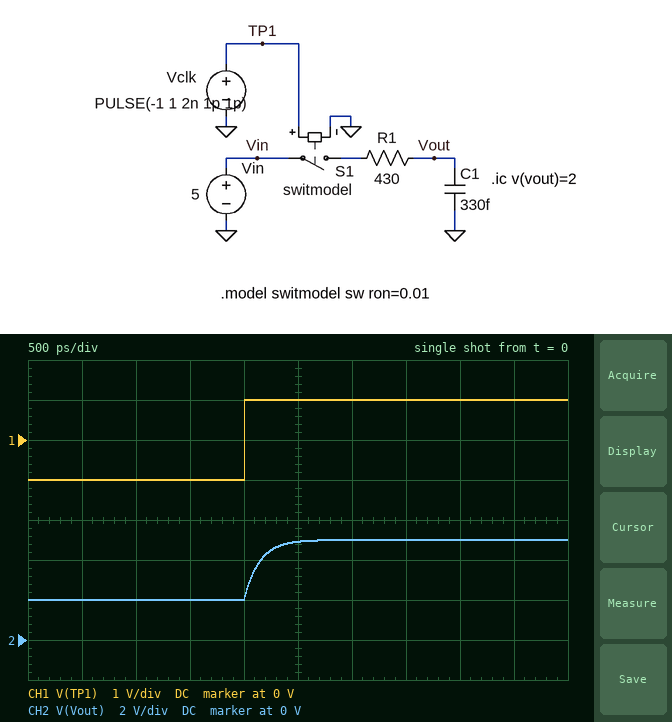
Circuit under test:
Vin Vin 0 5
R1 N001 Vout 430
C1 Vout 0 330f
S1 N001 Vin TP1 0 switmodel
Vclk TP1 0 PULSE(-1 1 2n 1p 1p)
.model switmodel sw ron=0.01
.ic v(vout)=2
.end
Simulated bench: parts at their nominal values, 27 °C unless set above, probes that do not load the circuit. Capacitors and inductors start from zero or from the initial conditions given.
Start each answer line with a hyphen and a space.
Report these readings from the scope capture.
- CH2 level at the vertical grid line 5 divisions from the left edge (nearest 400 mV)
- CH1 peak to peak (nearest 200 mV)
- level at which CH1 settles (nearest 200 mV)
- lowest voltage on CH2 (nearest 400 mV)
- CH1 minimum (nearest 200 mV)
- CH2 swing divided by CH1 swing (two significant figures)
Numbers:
- 4.8 V
- 2.0 V
- 1.0 V
- 2.0 V
- -1.0 V
- 1.5
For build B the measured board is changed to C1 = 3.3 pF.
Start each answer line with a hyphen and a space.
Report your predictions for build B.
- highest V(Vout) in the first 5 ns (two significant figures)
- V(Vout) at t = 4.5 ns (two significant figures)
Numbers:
- 4.6 V
- 4.5 V
